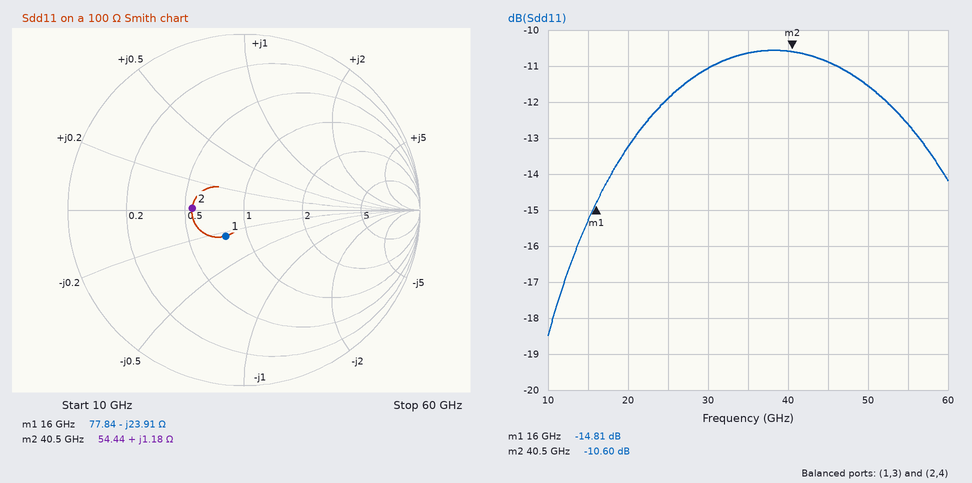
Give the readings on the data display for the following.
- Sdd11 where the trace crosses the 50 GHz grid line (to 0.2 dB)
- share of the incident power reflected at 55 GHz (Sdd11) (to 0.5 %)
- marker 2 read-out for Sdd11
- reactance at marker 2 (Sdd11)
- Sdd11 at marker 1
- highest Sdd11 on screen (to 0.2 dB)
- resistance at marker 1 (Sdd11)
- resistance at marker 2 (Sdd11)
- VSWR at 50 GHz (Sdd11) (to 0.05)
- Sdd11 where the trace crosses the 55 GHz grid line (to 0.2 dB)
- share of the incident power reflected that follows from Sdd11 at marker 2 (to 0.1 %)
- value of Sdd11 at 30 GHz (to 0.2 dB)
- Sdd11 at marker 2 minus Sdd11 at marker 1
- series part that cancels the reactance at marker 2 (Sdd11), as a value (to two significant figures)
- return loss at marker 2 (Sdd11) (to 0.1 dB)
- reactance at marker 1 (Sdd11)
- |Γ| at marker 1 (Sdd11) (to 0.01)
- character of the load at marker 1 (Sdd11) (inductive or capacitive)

-11.6 dB
5.5 %
-10.60 dB
+1.18 Ω
-14.81 dB
-10.6 dB
77.84 Ω
54.44 Ω
1.70
-12.6 dB
8.7 %
-11.0 dB
4.21 dB
3.3 pF
10.6 dB
-23.91 Ω
0.18
capacitive
